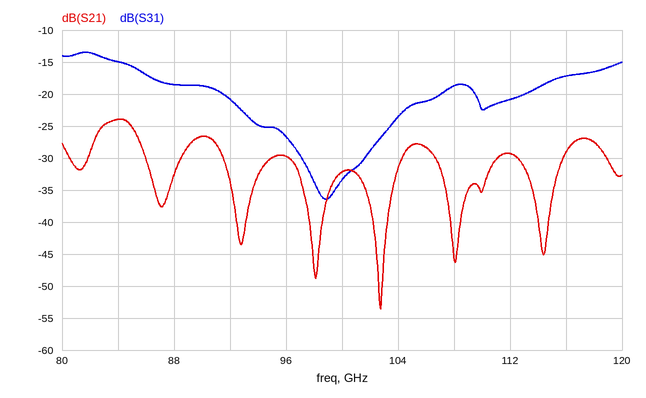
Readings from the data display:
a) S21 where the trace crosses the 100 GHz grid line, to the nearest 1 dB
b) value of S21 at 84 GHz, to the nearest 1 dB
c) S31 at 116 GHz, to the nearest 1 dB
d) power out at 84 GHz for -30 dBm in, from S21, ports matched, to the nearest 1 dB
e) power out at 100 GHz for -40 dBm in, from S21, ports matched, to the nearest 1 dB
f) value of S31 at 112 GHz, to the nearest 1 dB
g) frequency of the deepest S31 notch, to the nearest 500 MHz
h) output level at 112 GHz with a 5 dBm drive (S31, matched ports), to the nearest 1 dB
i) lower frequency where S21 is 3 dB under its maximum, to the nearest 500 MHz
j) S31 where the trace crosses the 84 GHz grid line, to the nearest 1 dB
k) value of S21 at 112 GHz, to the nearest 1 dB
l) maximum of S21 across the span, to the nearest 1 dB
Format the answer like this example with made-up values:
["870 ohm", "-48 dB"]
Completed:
["-32 dB", "-24 dB", "-17 dB", "-54 dBm", "-72 dBm", "-21 dB", "99.0 GHz", "-16 dBm", "82.5 GHz", "-15 dB", "-29 dB", "-24 dB"]
